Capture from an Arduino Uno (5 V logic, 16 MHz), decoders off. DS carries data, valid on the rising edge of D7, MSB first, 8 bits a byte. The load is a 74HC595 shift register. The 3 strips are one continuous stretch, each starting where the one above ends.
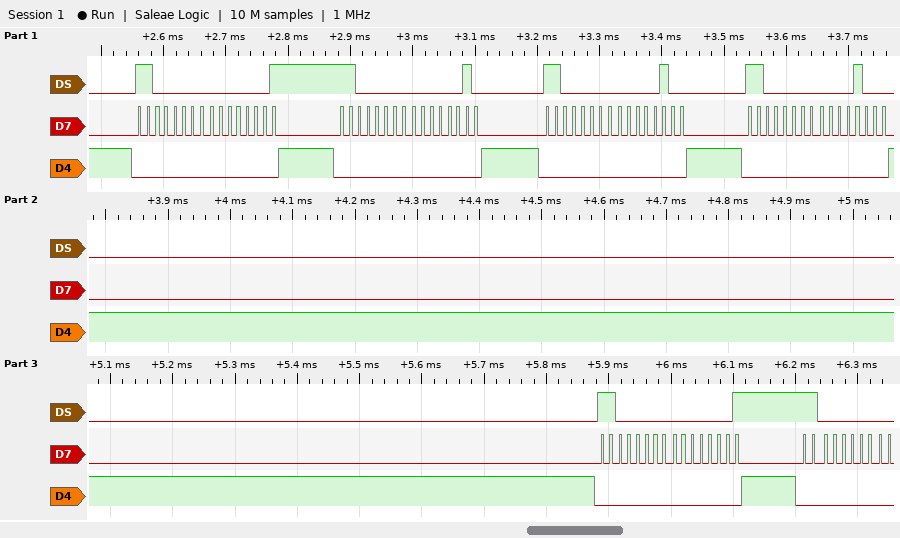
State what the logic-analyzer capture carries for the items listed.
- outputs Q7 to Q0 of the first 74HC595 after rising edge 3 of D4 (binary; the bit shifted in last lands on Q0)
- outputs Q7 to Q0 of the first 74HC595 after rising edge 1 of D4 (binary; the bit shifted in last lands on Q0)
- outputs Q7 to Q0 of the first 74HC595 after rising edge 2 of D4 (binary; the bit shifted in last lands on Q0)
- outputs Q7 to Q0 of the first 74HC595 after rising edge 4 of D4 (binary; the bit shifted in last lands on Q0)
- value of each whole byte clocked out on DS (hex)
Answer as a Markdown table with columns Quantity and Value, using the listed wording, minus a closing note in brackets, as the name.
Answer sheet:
| Quantity | Value |
|---|---|
| outputs Q7 to Q0 of the first 74HC595 after rising edge 3 of D4 | 00000100 |
| outputs Q7 to Q0 of the first 74HC595 after rising edge 1 of D4 | 00000001 |
| outputs Q7 to Q0 of the first 74HC595 after rising edge 2 of D4 | 00000010 |
| outputs Q7 to Q0 of the first 74HC595 after rising edge 4 of D4 | 00001000 |
| value of each whole byte clocked out on DS | C0 01 C0 02 C0 04 C0 08 C0 01 C0 |
